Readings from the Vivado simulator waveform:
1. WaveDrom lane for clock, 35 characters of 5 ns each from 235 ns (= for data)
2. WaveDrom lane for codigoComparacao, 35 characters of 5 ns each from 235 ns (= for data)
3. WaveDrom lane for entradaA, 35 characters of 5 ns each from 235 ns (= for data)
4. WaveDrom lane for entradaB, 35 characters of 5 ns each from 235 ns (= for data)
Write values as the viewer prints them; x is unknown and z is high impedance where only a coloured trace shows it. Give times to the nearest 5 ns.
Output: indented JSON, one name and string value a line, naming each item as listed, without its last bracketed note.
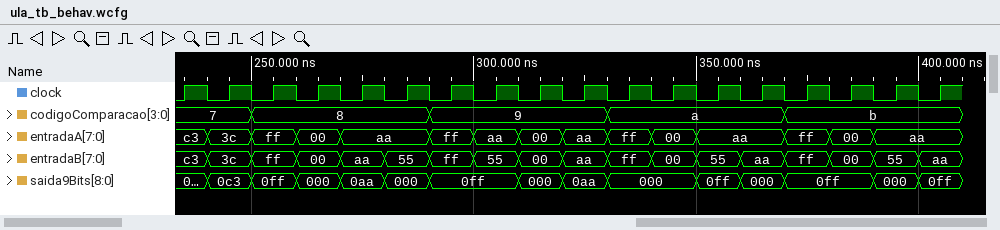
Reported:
{
  "WaveDrom lane for clock, 35 characters of 5 ns each from 235 ns": "{name: 'clock', wave: '10101010101010101010101010101010101'}",
  "WaveDrom lane for codigoComparacao, 35 characters of 5 ns each from 235 ns": "{name: 'codigoComparacao', wave: '=..=.......=.......=.......=.......', data: '7 8 9 a b'}",
  "WaveDrom lane for entradaA, 35 characters of 5 ns each from 235 ns": "{name: 'entradaA', wave: '==.=.=.=...=.=.=.=.=.=.=...=.=.=...', data: 'c3 3c ff 00 aa ff aa 00 aa ff 00 aa ff 00 aa'}",
  "WaveDrom lane for entradaB, 35 characters of 5 ns each from 235 ns": "{name: 'entradaB', wave: '==.=.=.=.=.=.=.=.=.=.=.=.=.=.=.=.=.', data: 'c3 3c ff 00 aa 55 ff 55 00 aa ff 00 55 aa ff 00 55 aa'}"
}
